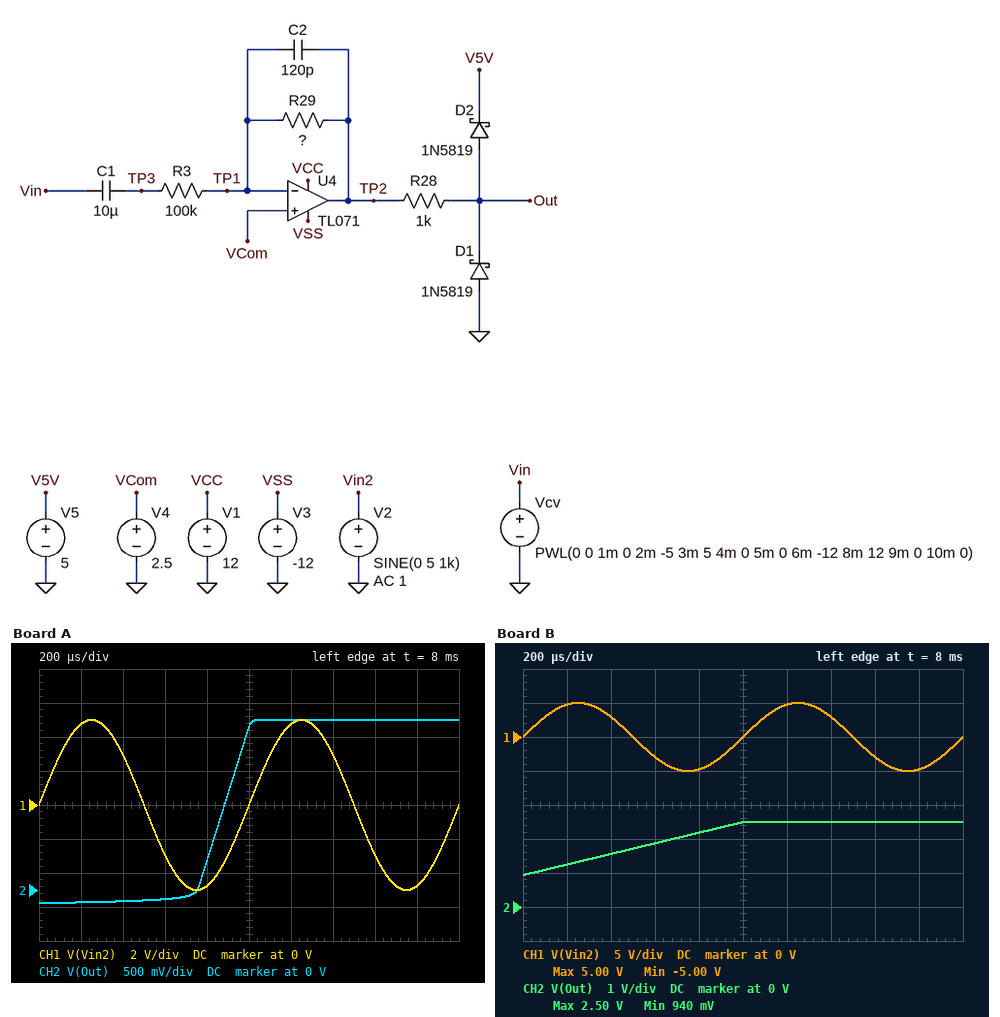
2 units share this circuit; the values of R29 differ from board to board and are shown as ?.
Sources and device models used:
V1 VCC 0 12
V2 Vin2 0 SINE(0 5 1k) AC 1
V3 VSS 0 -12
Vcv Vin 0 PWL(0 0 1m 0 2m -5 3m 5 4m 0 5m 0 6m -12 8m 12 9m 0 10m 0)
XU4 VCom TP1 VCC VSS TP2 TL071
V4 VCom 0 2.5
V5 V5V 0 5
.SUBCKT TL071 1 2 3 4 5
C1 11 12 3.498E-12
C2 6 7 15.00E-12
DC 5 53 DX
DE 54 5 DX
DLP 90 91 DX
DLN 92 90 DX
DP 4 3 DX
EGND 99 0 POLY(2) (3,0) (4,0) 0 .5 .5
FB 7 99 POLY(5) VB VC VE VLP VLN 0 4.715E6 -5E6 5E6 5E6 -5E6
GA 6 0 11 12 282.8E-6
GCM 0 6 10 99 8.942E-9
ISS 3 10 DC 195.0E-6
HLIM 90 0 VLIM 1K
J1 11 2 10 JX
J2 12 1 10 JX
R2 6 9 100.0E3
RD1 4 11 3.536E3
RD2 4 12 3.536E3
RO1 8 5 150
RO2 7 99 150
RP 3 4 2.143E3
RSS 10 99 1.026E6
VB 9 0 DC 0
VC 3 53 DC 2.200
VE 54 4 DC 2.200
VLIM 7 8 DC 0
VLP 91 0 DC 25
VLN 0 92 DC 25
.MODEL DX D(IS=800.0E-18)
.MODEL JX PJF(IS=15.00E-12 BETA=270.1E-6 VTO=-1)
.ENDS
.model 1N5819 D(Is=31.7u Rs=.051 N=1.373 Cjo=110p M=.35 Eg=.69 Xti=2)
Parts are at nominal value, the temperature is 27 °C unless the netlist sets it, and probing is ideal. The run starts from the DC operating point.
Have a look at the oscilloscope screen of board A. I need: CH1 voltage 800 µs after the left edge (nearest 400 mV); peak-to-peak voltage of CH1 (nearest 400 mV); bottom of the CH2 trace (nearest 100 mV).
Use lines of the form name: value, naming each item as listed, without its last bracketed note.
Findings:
CH1 voltage 800 µs after the left edge: -4.8 V
peak-to-peak voltage of CH1: 10.0 V
bottom of the CH2 trace: -200 mV
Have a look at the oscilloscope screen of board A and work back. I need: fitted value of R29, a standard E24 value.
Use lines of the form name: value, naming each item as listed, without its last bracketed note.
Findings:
fitted value of R29, a standard E24 value: 82 kΩ
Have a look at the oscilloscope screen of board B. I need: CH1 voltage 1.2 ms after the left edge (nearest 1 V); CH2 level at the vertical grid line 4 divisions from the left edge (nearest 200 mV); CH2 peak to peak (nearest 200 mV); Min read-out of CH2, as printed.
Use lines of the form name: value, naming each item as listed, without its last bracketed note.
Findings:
CH1 voltage 1.2 ms after the left edge: 5 V
CH2 level at the vertical grid line 4 divisions from the left edge: 2.2 V
CH2 peak to peak: 1.6 V
Min read-out of CH2, as printed: 940 mV
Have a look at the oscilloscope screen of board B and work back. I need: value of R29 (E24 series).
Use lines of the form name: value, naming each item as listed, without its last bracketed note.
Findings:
value of R29: 13 kΩ
